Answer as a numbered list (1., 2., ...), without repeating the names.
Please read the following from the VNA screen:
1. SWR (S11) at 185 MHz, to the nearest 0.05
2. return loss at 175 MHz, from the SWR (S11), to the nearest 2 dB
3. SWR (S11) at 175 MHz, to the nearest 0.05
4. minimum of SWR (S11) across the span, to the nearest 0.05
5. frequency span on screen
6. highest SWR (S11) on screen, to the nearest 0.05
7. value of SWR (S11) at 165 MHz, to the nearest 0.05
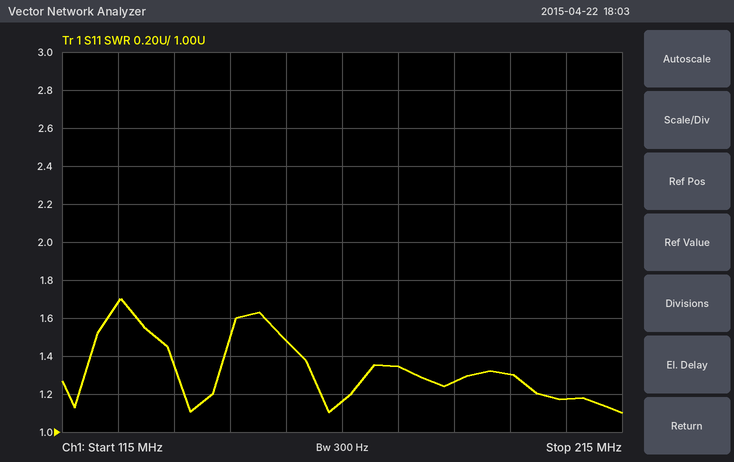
1. 1.25
2. 16 dB
3. 1.35
4. 1.10
5. 100 MHz
6. 1.70
7. 1.15
